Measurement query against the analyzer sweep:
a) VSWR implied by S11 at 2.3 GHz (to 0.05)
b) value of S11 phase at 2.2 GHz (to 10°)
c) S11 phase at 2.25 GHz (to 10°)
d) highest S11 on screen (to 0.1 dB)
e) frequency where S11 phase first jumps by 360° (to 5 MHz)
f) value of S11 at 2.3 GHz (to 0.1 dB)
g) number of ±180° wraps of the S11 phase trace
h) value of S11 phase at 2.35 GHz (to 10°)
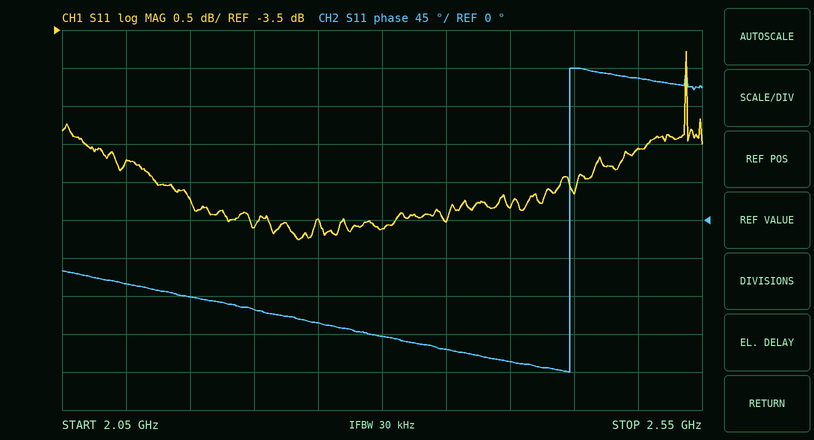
2.95
-110°
-120°
-3.8 dB
2.445 GHz
-6.1 dB
1
-150°
